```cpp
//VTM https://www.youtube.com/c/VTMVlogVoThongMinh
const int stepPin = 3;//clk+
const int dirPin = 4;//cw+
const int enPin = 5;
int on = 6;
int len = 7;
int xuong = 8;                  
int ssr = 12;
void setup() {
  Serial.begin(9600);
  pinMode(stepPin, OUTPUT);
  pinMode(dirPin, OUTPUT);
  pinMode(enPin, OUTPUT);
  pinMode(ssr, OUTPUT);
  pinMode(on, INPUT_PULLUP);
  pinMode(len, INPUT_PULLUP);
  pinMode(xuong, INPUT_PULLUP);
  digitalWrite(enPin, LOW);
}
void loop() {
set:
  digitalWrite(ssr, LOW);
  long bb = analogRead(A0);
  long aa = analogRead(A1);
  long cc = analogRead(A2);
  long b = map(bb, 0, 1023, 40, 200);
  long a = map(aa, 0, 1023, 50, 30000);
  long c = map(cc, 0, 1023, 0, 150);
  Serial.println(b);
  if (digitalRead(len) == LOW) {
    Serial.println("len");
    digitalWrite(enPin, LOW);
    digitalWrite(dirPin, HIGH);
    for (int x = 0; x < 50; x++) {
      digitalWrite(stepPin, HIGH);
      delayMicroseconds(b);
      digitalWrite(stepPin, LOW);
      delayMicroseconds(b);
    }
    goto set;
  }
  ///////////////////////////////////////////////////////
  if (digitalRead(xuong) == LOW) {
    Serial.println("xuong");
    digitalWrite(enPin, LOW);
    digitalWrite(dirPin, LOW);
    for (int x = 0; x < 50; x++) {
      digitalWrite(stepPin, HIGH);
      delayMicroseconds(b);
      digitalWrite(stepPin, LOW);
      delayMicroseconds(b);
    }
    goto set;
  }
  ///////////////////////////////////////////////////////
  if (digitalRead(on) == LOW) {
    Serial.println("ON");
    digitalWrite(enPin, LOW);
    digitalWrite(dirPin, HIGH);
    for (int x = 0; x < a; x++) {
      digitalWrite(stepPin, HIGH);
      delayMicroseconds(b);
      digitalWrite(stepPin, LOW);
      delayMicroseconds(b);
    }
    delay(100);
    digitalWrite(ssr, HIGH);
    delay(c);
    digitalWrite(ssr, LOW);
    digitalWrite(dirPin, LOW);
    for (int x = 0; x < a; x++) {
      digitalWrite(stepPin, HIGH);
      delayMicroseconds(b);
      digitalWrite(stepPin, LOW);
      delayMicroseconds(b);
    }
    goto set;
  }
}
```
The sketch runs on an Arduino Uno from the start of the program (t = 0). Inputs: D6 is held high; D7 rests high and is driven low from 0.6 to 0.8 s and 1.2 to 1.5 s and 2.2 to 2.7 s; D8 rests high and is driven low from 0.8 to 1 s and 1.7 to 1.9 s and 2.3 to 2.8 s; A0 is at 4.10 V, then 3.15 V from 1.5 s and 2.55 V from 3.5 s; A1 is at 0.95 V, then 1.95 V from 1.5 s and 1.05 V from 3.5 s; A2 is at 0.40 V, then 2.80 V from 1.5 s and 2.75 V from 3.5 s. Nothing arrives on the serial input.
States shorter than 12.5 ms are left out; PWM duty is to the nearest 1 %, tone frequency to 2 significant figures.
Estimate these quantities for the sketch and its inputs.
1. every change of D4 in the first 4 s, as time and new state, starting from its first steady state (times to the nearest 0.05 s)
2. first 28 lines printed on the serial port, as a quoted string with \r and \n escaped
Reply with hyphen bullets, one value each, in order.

- 0 s low; 0.6 s high; 0.8 s low; 1.2 s high; 1.7 s low; 2.2 s high; 2.7 s low
- "171\r\n171\r\n171\r\n171\r\n171\r\n171\r\n171\r\n171\r\n171\r\n171\r\n171\r\n171\r\n171\r\n171\r\n171\r\n171\r\n171\r\n171\r\n171\r\n171\r\n171\r\n171\r\n171\r\n171\r\n171\r\n171\r\n171\r\n171\r\n"
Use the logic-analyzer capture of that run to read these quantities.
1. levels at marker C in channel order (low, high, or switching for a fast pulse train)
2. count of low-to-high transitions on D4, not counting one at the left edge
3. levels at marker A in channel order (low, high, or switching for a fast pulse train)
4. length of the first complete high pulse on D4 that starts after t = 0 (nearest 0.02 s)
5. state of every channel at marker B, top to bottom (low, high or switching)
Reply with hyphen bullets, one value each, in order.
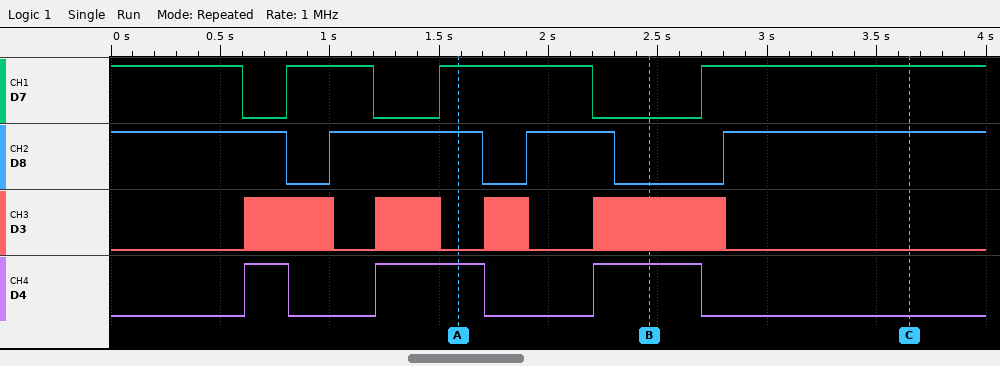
- D7 high, D8 high, D3 low, D4 low
- 3
- D7 high, D8 high, D3 low, D4 high
- 0.20 s
- D7 low, D8 low, D3 switching, D4 high
